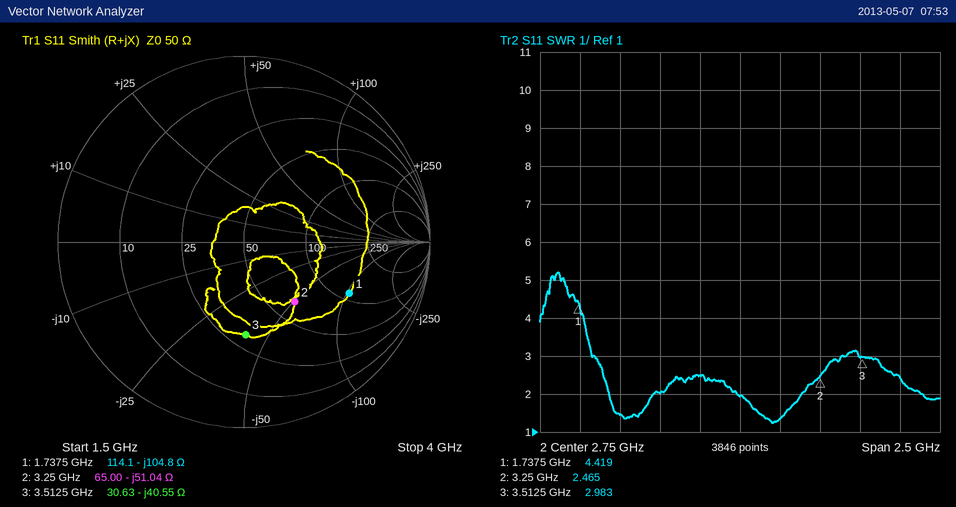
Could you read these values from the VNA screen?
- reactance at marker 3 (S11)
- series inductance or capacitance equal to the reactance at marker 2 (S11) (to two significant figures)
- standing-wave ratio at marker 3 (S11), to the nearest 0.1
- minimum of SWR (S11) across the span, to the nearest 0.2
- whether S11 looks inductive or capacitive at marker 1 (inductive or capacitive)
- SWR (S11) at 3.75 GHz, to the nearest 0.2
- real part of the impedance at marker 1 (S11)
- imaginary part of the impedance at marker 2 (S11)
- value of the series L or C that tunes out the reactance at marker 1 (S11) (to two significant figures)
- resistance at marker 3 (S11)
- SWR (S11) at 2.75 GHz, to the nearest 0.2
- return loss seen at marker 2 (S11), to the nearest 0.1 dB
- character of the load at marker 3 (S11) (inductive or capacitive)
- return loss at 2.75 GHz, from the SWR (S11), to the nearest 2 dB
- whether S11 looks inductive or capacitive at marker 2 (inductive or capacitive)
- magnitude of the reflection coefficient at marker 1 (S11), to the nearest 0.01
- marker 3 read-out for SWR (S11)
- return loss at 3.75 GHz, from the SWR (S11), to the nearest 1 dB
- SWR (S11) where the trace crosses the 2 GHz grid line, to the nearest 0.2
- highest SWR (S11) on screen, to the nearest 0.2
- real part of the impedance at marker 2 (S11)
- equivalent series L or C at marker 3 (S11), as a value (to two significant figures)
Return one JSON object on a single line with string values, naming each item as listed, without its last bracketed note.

{"reactance at marker 3": "-40.55 Ω", "series inductance or capacitance equal to the reactance at marker 2 (S11)": "960 fF", "standing-wave ratio at marker 3 (S11), to the nearest 0.1": "3.0", "minimum of SWR (S11) across the span, to the nearest 0.2": "1.2", "whether S11 looks inductive or capacitive at marker 1": "capacitive", "SWR (S11) at 3.75 GHz, to the nearest 0.2": "2.4", "real part of the impedance at marker 1": "114.1 Ω", "imaginary part of the impedance at marker 2": "-51.04 Ω", "value of the series L or C that tunes out the reactance at marker 1 (S11)": "9.6 nH", "resistance at marker 3": "30.63 Ω", "SWR (S11) at 2.75 GHz, to the nearest 0.2": "2.0", "return loss seen at marker 2 (S11), to the nearest 0.1 dB": "7.5 dB", "character of the load at marker 3 (S11)": "capacitive", "return loss at 2.75 GHz, from the SWR (S11), to the nearest 2 dB": "10 dB", "whether S11 looks inductive or capacitive at marker 2": "capacitive", "magnitude of the reflection coefficient at marker 1 (S11), to the nearest 0.01": "0.63", "marker 3 read-out for SWR": "2.983", "return loss at 3.75 GHz, from the SWR (S11), to the nearest 1 dB": "8 dB", "SWR (S11) where the trace crosses the 2 GHz grid line, to the nearest 0.2": "1.4", "highest SWR (S11) on screen, to the nearest 0.2": "5.2", "real part of the impedance at marker 2": "65.00 Ω", "equivalent series L or C at marker 3 (S11), as a value": "1.1 pF"}
